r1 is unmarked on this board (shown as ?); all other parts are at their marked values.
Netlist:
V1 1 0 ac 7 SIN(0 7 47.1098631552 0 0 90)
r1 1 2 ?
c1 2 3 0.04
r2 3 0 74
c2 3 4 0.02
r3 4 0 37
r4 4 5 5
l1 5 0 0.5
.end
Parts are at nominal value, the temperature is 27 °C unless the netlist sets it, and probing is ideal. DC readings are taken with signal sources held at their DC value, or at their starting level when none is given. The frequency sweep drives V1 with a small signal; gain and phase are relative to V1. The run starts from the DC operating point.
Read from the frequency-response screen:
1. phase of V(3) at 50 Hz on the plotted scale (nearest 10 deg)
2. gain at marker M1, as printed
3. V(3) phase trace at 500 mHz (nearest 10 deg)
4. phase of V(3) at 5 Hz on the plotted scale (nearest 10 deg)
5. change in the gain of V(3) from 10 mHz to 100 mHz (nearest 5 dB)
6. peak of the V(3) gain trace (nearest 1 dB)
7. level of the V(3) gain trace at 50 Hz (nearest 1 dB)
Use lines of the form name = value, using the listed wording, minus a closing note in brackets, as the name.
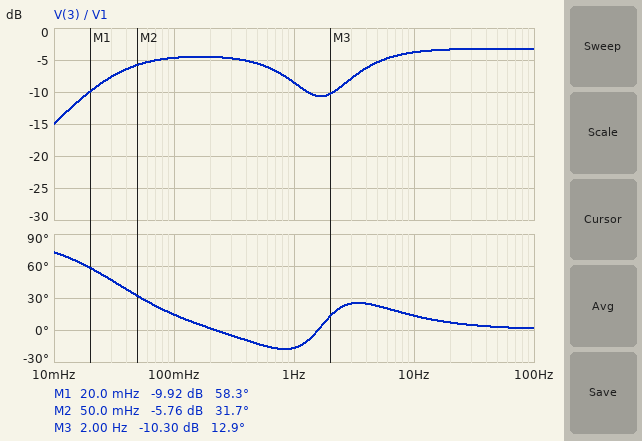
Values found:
phase of V(3) at 50 Hz on the plotted scale = 0 deg
gain at marker M1, as printed = -9.92 dB
V(3) phase trace at 500 mHz = -10 deg
phase of V(3) at 5 Hz on the plotted scale = 20 deg
change in the gain of V(3) from 10 mHz to 100 mHz = 10 dB
peak of the V(3) gain trace = -3 dB
level of the V(3) gain trace at 50 Hz = -3 dB
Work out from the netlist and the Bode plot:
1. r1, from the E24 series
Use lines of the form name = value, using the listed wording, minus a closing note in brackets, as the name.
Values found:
r1, from the E24 series = 11 Ω
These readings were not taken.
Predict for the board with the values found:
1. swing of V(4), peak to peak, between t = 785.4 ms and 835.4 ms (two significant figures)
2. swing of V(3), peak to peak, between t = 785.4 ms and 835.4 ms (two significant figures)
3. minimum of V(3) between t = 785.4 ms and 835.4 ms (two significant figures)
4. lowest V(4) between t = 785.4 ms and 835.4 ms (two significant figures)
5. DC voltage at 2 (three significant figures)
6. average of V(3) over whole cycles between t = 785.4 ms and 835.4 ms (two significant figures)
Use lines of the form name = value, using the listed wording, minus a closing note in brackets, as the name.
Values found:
swing of V(4), peak to peak, between t = 785.4 ms and 835.4 ms = 9.7 V
swing of V(3), peak to peak, between t = 785.4 ms and 835.4 ms = 9.7 V
minimum of V(3) between t = 785.4 ms and 835.4 ms = -8.6 V
lowest V(4) between t = 785.4 ms and 835.4 ms = -4.8 V
DC voltage at 2 = 7.00 V
average of V(3) over whole cycles between t = 785.4 ms and 835.4 ms = -3.7 V
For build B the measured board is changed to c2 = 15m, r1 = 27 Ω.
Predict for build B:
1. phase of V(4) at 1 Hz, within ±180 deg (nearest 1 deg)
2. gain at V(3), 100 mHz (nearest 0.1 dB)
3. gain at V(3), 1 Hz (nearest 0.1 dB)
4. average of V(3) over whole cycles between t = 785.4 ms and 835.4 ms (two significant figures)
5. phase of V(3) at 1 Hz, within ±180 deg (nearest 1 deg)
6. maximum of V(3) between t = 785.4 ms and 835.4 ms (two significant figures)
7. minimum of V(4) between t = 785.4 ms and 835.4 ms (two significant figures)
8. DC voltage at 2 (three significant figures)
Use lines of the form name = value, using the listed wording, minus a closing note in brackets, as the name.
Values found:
phase of V(4) at 1 Hz, within ±180 deg = 53 deg
gain at V(3), 100 mHz = -5.0 dB
gain at V(3), 1 Hz = -11.7 dB
average of V(3) over whole cycles between t = 785.4 ms and 835.4 ms = -3.5 V
phase of V(3) at 1 Hz, within ±180 deg = -36 deg
maximum of V(3) between t = 785.4 ms and 835.4 ms = -210 mV
minimum of V(4) between t = 785.4 ms and 835.4 ms = -3.3 V
DC voltage at 2 = 7.00 V
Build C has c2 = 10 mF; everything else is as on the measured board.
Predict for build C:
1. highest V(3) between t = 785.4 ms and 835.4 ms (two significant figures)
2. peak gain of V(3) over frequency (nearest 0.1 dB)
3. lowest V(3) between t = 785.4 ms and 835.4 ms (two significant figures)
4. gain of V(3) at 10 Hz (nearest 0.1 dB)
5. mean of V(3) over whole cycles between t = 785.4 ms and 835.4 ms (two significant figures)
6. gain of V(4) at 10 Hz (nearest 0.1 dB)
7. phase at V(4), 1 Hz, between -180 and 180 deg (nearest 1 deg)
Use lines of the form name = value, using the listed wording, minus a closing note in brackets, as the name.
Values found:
highest V(3) between t = 785.4 ms and 835.4 ms = 590 mV
peak gain of V(3) over frequency = -3.0 dB
lowest V(3) between t = 785.4 ms and 835.4 ms = -9.1 V
gain of V(3) at 10 Hz = -3.9 dB
mean of V(3) over whole cycles between t = 785.4 ms and 835.4 ms = -4.3 V
gain of V(4) at 10 Hz = -3.5 dB
phase at V(4), 1 Hz, between -180 and 180 deg = 80 deg
